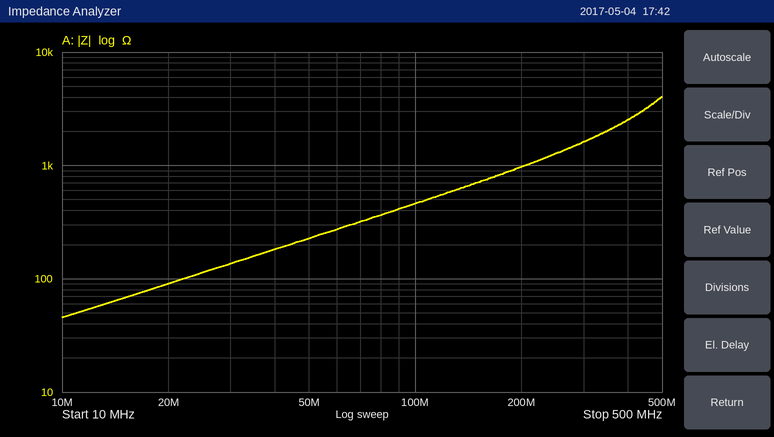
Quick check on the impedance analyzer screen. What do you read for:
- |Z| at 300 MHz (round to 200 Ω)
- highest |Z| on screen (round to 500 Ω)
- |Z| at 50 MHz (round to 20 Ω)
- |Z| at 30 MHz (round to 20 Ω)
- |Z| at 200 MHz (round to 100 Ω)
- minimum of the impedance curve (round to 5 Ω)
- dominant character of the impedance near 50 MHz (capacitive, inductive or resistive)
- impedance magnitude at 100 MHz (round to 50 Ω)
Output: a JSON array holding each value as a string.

["1.6 kΩ", "4.0 kΩ", "220 Ω", "140 Ω", "1.0 kΩ", "45 Ω", "inductive", "450 Ω"]
